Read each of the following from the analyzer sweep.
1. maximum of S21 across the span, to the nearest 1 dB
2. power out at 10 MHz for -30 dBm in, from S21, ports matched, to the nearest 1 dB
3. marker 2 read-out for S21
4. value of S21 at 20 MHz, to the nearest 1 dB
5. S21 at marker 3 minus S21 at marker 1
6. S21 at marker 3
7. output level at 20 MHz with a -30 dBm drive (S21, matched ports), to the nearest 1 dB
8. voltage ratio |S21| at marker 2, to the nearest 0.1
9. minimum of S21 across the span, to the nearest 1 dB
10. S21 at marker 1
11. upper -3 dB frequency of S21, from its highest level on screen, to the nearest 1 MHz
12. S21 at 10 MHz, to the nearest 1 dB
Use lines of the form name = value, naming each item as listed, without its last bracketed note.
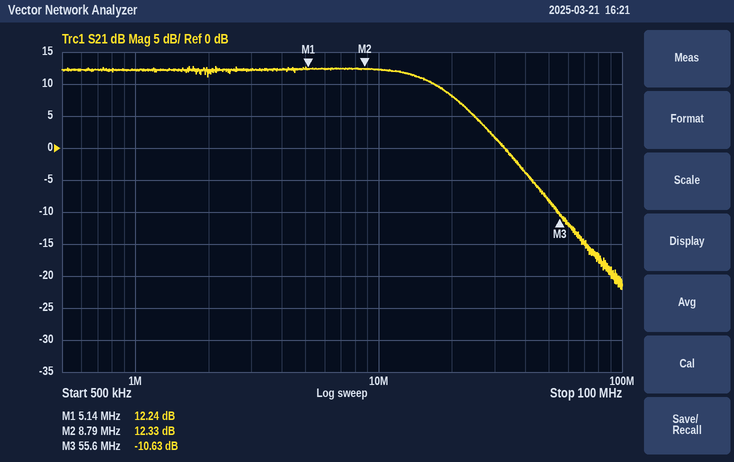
maximum of S21 across the span, to the nearest 1 dB = 13 dB
power out at 10 MHz for -30 dBm in, from S21, ports matched, to the nearest 1 dB = -18 dBm
marker 2 read-out for S21 = 12.33 dB
value of S21 at 20 MHz, to the nearest 1 dB = 8 dB
S21 at marker 3 minus S21 at marker 1 = -22.87 dB
S21 at marker 3 = -10.63 dB
output level at 20 MHz with a -30 dBm drive (S21, matched ports), to the nearest 1 dB = -22 dBm
voltage ratio |S21| at marker 2, to the nearest 0.1 = 4.1
minimum of S21 across the span, to the nearest 1 dB = -22 dB
S21 at marker 1 = 12.24 dB
upper -3 dB frequency of S21, from its highest level on screen, to the nearest 1 MHz = 17 MHz
S21 at 10 MHz, to the nearest 1 dB = 12 dB
